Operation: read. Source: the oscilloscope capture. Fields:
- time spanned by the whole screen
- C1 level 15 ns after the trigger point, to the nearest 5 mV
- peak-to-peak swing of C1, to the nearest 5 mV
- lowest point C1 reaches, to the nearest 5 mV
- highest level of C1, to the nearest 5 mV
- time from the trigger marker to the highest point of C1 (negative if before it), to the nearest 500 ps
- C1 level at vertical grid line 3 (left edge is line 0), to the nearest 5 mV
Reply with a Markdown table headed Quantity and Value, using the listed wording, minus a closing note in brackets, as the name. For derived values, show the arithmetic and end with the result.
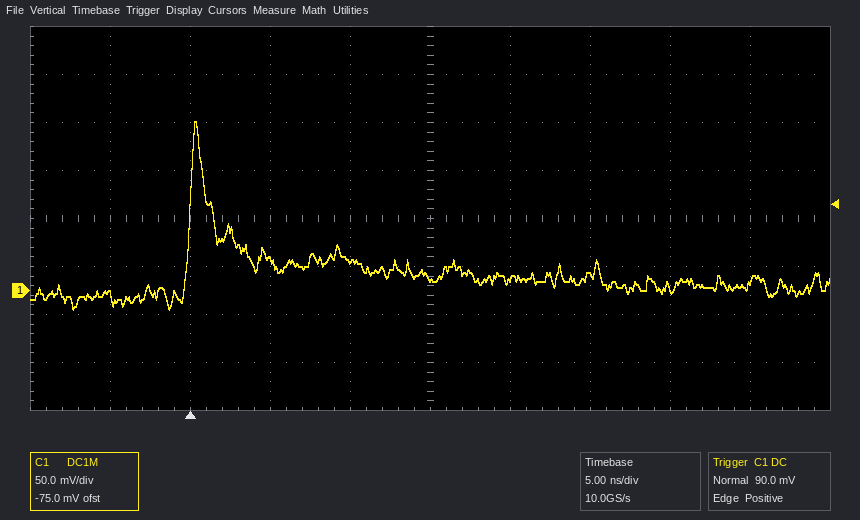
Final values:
| Quantity | Value |
|---|---|
| time spanned by the whole screen | 50 ns |
| C1 level 15 ns after the trigger point, to the nearest 5 mV | 15 mV |
| peak-to-peak swing of C1, to the nearest 5 mV | 175 mV − (-20 mV) = 195 mV |
| lowest point C1 reaches, to the nearest 5 mV | -20 mV |
| highest level of C1, to the nearest 5 mV | 175 mV |
| time from the trigger marker to the highest point of C1 (negative if before it), to the nearest 500 ps | +500 ps |
| C1 level at vertical grid line 3 (left edge is line 0), to the nearest 5 mV | 30 mV |
